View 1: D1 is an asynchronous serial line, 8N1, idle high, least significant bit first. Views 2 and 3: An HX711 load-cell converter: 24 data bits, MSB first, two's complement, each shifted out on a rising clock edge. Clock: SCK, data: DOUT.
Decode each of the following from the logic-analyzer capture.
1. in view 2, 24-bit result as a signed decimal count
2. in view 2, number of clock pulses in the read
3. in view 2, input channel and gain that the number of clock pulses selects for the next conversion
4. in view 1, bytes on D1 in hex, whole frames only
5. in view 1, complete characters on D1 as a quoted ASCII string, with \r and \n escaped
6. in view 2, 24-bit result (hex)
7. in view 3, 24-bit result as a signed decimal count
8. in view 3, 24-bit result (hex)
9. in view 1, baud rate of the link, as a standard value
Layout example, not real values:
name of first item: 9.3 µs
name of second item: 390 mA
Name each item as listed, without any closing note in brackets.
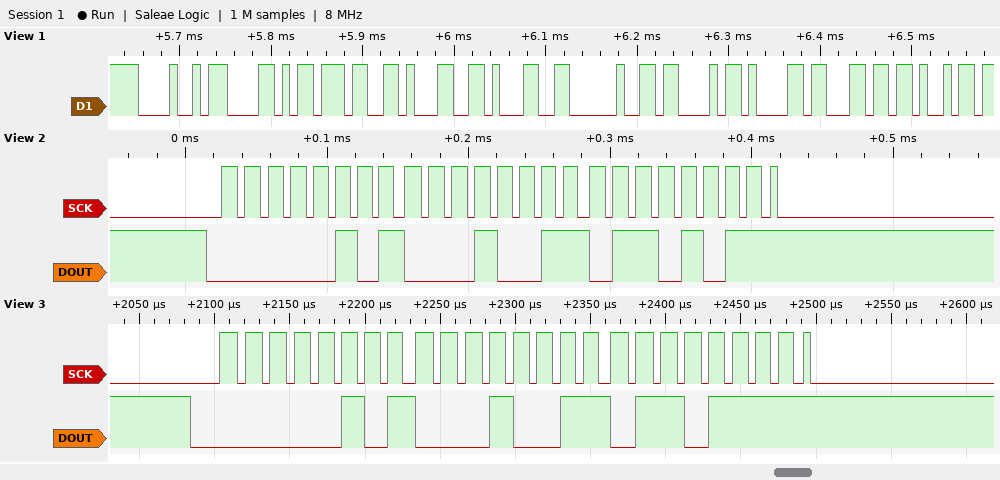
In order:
in view 2, 24-bit result as a signed decimal count: 332651
in view 2, number of clock pulses in the read: 25
in view 2, input channel and gain that the number of clock pulses selects for the next conversion: channel A, gain 128
in view 1, bytes on D1 in hex, whole frames only: 48 58 37 31 31 20 43 61 6C 69
in view 1, complete characters on D1 as a quoted ASCII string, with \r and \n escaped: "HX711 Cali"
in view 2, 24-bit result: 0x05136B
in view 3, 24-bit result as a signed decimal count: 332655
in view 3, 24-bit result: 0x05136F
in view 1, baud rate of the link, as a standard value: 115200 baud
